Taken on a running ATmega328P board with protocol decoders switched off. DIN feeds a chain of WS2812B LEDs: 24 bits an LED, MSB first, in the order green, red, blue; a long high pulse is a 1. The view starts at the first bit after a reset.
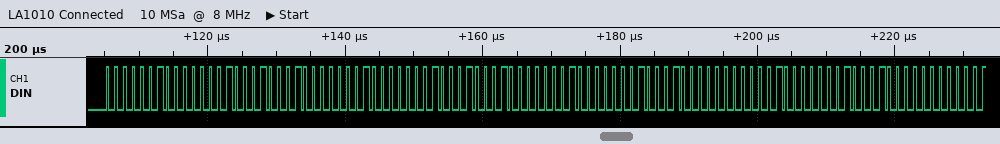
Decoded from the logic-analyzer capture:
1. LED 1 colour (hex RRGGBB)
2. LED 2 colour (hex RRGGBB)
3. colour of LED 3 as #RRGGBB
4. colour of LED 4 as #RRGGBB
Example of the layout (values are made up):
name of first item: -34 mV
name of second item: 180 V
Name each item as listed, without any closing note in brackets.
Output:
LED 1 colour: #020222
LED 2 colour: #020222
colour of LED 3 as #RRGGBB: #020220
colour of LED 4 as #RRGGBB: #020220
